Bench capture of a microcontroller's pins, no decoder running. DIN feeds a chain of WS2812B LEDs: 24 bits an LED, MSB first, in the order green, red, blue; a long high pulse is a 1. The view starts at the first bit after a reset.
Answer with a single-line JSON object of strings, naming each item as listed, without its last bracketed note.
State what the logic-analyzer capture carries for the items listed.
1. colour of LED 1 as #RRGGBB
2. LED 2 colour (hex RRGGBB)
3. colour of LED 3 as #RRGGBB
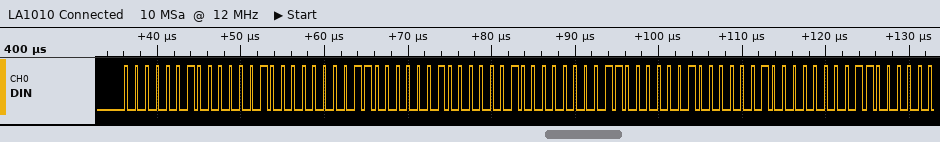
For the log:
{"colour of LED 1 as #RRGGBB": "#040203", "LED 2 colour": "#040203", "colour of LED 3 as #RRGGBB": "#040203"}
